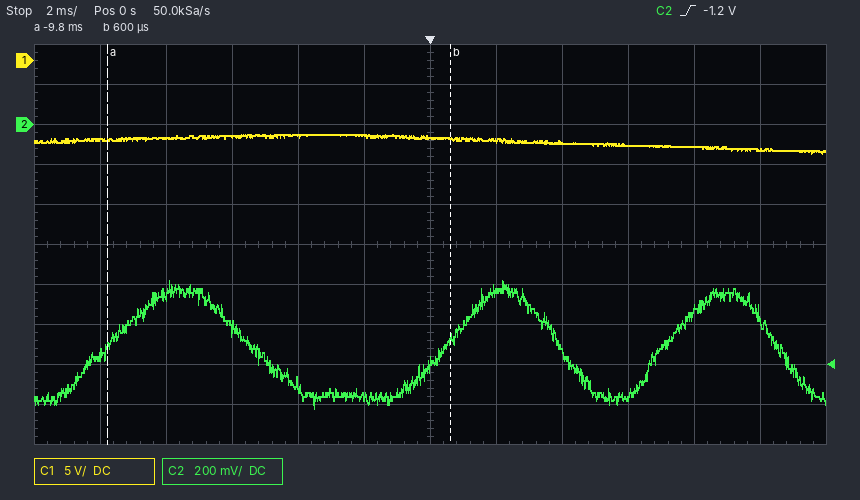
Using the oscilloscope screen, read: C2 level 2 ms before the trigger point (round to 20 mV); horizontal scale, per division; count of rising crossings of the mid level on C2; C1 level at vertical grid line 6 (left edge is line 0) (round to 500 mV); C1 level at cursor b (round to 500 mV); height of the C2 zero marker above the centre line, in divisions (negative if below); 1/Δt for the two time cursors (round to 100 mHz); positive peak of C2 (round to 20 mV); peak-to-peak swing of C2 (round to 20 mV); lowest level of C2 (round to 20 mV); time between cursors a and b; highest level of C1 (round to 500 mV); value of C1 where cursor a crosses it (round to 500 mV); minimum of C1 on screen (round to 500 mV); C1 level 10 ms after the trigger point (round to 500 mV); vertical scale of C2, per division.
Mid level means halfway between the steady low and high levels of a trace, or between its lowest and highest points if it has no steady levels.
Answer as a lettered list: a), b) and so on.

a) -1.36 V
b) 2 ms
c) 3
d) -9.5 V
e) -10.0 V
f) +3.0 div
g) 96.2 Hz
h) -780 mV
i) 640 mV
j) -1.42 V
k) 10.4 ms
l) -9.0 V
m) -10.0 V
n) -11.5 V
o) -11.0 V
p) 200 mV
